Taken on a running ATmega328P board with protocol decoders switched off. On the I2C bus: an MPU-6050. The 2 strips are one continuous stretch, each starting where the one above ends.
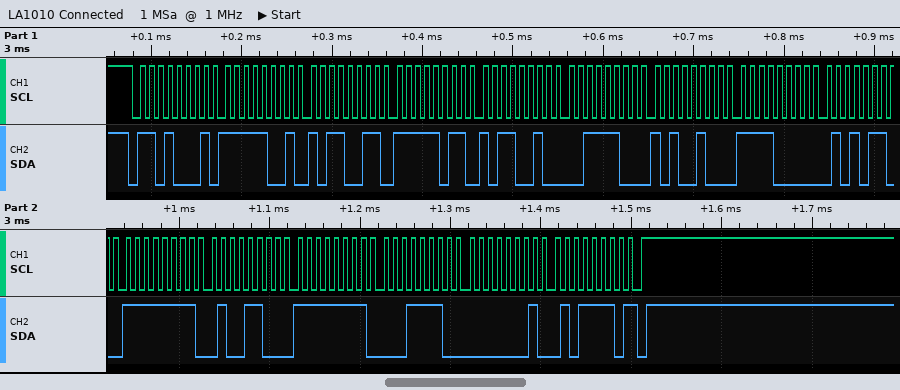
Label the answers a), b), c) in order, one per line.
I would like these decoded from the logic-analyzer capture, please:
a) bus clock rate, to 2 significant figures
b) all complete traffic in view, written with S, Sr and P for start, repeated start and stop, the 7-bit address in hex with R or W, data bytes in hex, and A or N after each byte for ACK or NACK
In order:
a) 100 kHz
b) S 68R A F9 A B3 A FB A B2 A 3C A A4 A F0 A 56 A FF A 4C A FF A 1E A 01 A 5E N P
